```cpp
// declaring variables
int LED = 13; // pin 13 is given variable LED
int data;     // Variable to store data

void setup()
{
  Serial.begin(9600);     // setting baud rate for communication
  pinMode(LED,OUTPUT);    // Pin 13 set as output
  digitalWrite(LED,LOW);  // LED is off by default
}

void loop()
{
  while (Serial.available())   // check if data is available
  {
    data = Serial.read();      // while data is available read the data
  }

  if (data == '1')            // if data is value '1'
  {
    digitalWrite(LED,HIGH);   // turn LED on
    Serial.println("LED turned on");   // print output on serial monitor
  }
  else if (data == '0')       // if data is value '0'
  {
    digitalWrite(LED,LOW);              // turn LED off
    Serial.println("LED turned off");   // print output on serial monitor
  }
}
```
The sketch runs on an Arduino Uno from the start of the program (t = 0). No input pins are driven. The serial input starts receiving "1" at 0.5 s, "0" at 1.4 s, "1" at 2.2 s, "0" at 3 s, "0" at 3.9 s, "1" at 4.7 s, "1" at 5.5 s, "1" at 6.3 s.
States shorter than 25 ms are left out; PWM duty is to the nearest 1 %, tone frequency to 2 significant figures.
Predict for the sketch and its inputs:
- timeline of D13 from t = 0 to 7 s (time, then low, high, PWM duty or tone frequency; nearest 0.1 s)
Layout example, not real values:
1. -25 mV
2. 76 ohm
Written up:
1. 0 s low; 0.5 s high; 1.4 s low; 2.2 s high; 3 s low; 4.7 s high
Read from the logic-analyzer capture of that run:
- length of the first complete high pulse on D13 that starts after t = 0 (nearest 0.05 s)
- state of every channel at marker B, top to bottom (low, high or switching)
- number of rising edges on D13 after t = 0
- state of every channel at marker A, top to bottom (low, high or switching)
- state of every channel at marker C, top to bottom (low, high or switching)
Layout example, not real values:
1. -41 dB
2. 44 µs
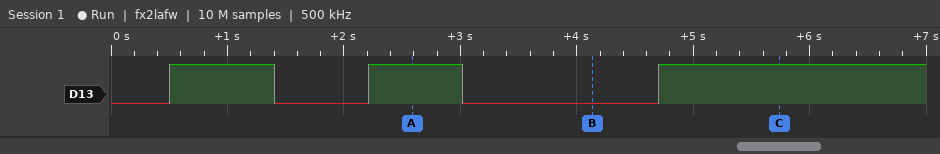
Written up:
1. 0.90 s
2. D13 low
3. 3
4. D13 high
5. D13 high
